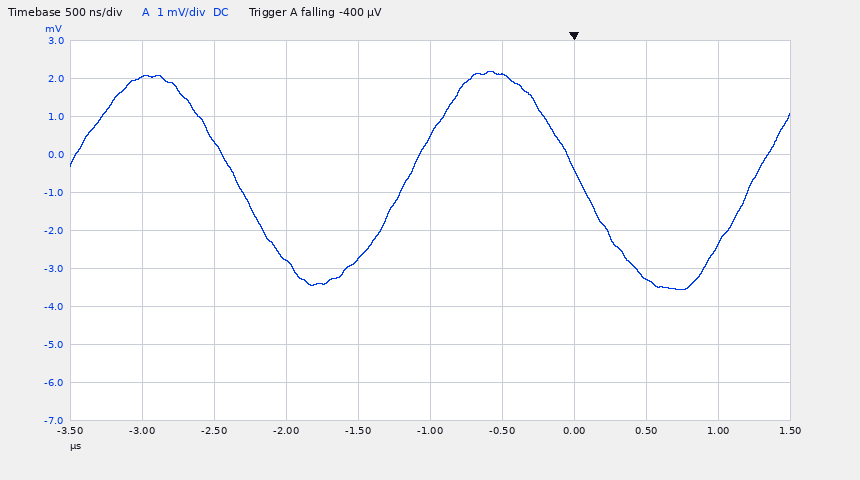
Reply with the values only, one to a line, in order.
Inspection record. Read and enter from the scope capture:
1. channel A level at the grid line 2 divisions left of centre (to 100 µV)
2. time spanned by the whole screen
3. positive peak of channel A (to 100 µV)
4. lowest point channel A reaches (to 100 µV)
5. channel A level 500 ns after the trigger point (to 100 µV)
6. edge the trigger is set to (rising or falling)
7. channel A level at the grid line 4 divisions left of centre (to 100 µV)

-2.8 mV
5 µs
2.2 mV
-3.6 mV
-3.3 mV
falling
2.0 mV
